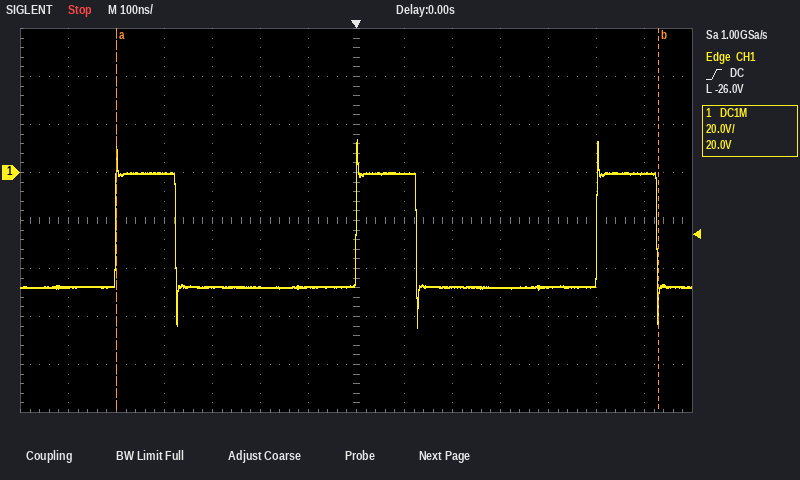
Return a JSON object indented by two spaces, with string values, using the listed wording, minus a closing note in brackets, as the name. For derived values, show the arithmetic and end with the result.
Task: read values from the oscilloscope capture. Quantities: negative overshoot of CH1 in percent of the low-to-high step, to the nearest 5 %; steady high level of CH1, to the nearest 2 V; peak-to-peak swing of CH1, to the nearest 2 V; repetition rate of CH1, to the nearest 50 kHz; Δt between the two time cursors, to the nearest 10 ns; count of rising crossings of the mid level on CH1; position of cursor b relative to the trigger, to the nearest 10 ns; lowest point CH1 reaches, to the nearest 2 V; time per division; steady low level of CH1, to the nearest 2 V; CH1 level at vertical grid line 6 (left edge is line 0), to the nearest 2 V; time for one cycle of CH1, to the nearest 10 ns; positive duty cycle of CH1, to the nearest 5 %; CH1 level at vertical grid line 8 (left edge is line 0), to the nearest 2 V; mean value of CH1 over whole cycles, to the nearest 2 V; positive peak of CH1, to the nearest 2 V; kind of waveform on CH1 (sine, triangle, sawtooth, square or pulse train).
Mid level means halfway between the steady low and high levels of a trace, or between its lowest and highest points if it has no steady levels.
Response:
{
  "negative overshoot of CH1 in percent of the low-to-high step, to the nearest 5 %": "35 %",
  "steady high level of CH1, to the nearest 2 V": "0 V",
  "peak-to-peak swing of CH1, to the nearest 2 V": "14 V − (-64 V) = 78 V",
  "repetition rate of CH1, to the nearest 50 kHz": "1 / 500 ns ≈ 2.00 MHz",
  "Δt between the two time cursors, to the nearest 10 ns": "1.13 µs",
  "count of rising crossings of the mid level on CH1": "3",
  "position of cursor b relative to the trigger, to the nearest 10 ns": "+630 ns",
  "lowest point CH1 reaches, to the nearest 2 V": "-64 V",
  "time per division": "100 ns",
  "steady low level of CH1, to the nearest 2 V": "-48 V",
  "CH1 level at vertical grid line 6 (left edge is line 0), to the nearest 2 V": "-48 V",
  "time for one cycle of CH1, to the nearest 10 ns": "500 ns",
  "positive duty cycle of CH1, to the nearest 5 %": "25 %",
  "CH1 level at vertical grid line 8 (left edge is line 0), to the nearest 2 V": "0 V",
  "mean value of CH1 over whole cycles, to the nearest 2 V": "-48 V + 0.25 × (0 V − (-48 V)) ≈ -36 V",
  "positive peak of CH1, to the nearest 2 V": "14 V",
  "kind of waveform on CH1": "pulse train"
}
